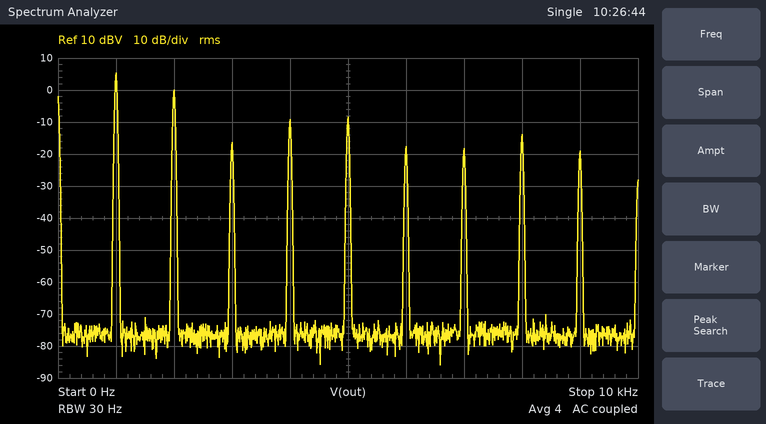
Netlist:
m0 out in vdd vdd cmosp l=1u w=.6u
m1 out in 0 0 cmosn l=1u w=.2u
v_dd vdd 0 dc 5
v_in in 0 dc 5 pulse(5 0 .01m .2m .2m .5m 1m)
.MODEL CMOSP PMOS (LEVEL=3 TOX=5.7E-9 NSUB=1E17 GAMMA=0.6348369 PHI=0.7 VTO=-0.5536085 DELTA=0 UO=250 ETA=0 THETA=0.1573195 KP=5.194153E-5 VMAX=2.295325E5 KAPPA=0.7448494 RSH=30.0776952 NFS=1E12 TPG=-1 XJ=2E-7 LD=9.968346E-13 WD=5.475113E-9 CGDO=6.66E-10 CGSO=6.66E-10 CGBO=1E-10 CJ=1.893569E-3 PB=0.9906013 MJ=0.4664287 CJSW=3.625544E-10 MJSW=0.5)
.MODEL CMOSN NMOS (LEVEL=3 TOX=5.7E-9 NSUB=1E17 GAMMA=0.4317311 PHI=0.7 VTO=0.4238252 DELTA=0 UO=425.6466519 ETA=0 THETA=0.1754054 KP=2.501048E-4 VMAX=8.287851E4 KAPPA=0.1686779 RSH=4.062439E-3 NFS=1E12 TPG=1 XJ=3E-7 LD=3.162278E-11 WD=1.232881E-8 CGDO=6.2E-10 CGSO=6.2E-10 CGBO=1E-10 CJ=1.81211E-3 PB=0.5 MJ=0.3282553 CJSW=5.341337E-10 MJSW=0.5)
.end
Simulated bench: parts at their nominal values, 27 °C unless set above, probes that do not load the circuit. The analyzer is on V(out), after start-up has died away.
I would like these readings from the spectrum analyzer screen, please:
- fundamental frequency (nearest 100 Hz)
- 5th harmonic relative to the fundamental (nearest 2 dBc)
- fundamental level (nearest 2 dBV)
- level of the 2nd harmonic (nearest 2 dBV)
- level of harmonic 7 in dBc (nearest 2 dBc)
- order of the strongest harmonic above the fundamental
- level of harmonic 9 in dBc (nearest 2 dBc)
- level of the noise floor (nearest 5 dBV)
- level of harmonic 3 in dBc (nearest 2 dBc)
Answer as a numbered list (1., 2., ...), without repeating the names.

1. 1.0 kHz
2. -14 dBc
3. 6 dBV
4. 0 dBV
5. -24 dBc
6. 2
7. -24 dBc
8. -75 dBV
9. -22 dBc
